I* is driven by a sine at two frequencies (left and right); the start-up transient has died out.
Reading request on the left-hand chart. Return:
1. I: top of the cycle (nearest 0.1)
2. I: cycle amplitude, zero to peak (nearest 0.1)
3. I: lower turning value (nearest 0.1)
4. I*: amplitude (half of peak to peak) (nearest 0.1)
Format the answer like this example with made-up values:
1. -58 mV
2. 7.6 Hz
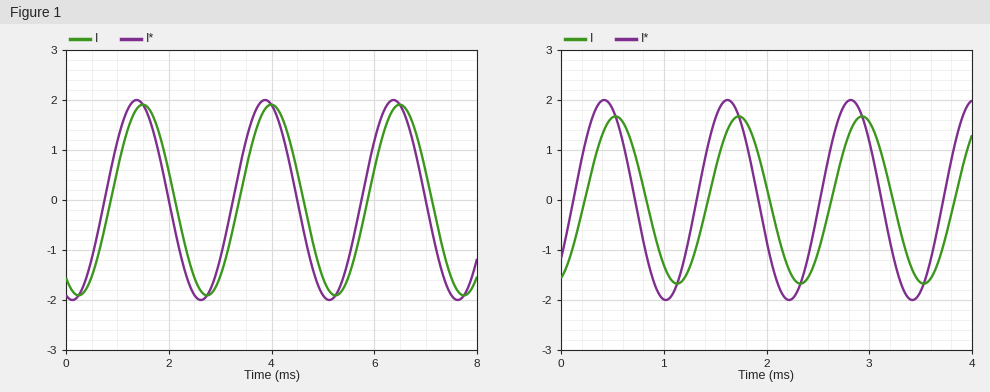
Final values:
1. 1.9
2. 1.9
3. -1.9
4. 2.0
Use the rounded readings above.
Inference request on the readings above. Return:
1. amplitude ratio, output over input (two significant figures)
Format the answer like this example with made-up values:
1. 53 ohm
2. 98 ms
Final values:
1. 0.95
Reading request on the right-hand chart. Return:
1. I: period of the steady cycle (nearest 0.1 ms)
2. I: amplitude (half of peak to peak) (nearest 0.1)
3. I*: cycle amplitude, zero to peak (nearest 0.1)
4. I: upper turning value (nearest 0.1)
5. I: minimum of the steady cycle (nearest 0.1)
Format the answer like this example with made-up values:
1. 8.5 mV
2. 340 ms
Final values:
1. 1.2 ms
2. 1.7
3. 2.0
4. 1.7
5. -1.7
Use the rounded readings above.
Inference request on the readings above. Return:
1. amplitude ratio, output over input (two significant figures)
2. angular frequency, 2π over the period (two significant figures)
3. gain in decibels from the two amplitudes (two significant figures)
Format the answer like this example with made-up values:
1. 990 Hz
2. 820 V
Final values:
1. 0.85
2. 5.2 rad/ms
3. -1.4 dB
